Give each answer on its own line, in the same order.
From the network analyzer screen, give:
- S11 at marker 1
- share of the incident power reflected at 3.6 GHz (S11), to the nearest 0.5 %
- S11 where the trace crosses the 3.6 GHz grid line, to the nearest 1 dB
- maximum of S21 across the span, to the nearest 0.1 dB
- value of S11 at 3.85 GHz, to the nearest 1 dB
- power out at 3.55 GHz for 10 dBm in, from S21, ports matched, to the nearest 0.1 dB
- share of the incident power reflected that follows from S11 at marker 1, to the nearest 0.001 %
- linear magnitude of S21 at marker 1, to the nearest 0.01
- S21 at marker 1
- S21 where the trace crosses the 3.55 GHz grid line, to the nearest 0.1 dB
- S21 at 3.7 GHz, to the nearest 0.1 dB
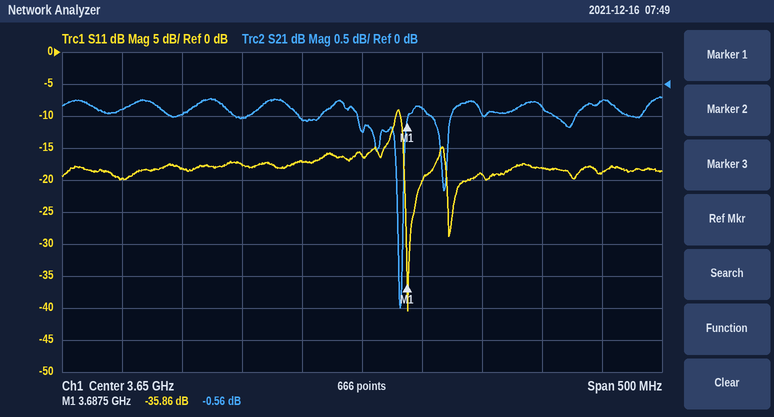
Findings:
-35.86 dB
2.0 %
-17 dB
-0.2 dB
-19 dB
9.5 dBm
0.026 %
0.94
-0.56 dB
-0.5 dB
-0.4 dB
